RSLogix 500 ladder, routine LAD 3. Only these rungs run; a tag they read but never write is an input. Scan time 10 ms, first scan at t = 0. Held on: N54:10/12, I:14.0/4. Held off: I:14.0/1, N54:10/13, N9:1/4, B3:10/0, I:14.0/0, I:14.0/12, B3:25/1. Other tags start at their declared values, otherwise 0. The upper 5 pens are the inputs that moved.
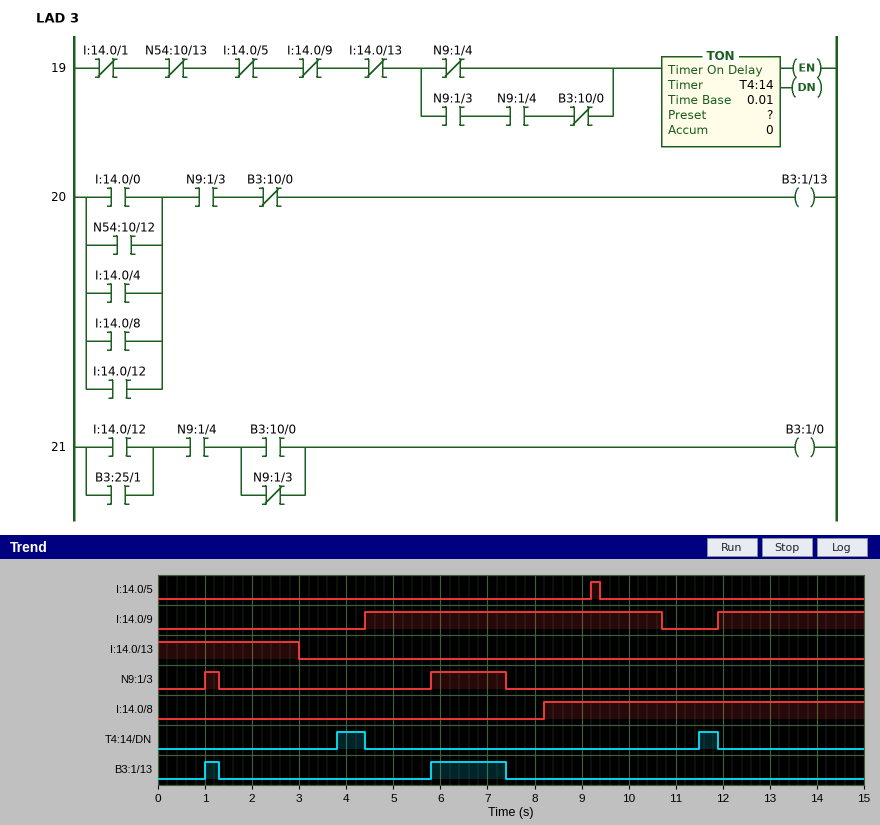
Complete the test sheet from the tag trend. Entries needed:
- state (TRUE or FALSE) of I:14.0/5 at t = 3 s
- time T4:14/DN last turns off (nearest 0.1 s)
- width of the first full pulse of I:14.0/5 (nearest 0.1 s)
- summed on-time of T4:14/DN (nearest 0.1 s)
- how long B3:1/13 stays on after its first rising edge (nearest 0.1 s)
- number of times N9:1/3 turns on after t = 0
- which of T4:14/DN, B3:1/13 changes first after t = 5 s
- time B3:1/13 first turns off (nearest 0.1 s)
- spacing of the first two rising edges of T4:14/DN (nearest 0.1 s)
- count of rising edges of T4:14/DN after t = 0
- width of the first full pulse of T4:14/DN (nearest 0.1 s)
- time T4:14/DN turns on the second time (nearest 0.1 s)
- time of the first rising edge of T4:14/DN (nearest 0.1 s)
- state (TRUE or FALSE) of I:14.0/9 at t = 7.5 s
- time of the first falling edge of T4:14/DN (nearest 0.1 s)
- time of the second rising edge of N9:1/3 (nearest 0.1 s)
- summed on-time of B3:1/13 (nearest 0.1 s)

FALSE
11.9 s
0.2 s
1.0 s
0.3 s
2
B3:1/13
1.3 s
7.7 s
2
0.6 s
11.5 s
3.8 s
TRUE
4.4 s
5.8 s
1.9 s
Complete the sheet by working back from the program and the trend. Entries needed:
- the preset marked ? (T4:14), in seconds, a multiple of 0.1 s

0.8 s
